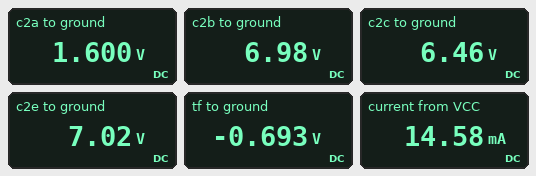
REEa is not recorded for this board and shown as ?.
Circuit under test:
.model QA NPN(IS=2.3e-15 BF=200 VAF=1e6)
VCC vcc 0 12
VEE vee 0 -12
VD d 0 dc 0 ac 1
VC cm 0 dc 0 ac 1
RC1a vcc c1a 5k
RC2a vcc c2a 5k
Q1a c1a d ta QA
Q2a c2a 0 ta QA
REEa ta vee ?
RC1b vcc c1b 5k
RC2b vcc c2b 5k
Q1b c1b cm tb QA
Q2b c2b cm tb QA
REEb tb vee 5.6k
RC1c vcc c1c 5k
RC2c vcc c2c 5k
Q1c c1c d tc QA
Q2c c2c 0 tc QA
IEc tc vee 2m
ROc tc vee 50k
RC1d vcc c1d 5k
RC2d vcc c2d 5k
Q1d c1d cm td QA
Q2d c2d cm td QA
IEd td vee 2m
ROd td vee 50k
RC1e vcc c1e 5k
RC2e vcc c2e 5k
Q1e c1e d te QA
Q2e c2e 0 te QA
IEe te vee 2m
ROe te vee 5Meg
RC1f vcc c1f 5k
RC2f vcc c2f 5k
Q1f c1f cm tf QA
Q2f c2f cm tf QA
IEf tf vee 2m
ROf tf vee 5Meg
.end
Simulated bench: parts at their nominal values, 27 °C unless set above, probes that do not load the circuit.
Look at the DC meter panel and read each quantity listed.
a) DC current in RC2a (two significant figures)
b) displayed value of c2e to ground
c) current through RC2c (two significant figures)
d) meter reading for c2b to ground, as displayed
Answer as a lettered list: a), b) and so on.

a) 2.1 mA
b) 7.02 V
c) 1.1 mA
d) 6.98 V
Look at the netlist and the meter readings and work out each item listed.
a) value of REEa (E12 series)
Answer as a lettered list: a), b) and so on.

a) 2.7 kΩ
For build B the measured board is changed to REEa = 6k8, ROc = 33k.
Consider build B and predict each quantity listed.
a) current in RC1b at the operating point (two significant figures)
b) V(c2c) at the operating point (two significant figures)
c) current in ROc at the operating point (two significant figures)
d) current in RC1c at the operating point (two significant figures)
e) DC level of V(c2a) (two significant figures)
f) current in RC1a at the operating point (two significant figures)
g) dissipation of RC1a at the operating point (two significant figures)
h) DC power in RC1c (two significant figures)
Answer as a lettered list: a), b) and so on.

a) 1.0 mA
b) 6.2 V
c) 340 µA
d) 1.2 mA
e) 7.9 V
f) 830 µA
g) 3.4 mW
h) 6.8 mW
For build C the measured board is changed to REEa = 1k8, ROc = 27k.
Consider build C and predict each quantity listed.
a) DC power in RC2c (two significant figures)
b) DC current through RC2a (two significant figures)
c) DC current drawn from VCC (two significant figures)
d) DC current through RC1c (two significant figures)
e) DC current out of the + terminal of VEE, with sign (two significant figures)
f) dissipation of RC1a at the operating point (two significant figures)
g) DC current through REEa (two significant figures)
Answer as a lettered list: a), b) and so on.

a) 7.2 mW
b) 2.5 mA
c) 16 mA
d) 1.2 mA
e) -17 mA
f) 32 mW
g) 6.3 mA
